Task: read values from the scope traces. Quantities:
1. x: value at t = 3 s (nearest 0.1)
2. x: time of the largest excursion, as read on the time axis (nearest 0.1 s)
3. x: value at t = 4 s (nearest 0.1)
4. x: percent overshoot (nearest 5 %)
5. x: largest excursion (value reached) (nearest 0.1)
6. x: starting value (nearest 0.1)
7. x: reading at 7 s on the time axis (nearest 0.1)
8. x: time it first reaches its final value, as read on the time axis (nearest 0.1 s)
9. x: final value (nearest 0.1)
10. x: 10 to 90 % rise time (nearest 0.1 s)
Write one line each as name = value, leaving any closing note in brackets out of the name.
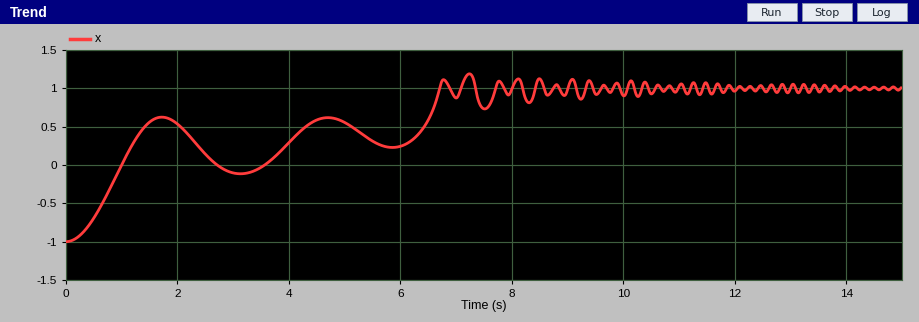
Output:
x: value at t = 3 s = -0.1
x: time of the largest excursion, as read on the time axis = 7.2 s
x: value at t = 4 s = 0.3
x: percent overshoot = 10 %
x: largest excursion (value reached) = 1.2
x: starting value = -1.0
x: reading at 7 s on the time axis = 0.9
x: time it first reaches its final value, as read on the time axis = 6.7 s
x: final value = 1.0
x: 10 to 90 % rise time = 6.2 s
